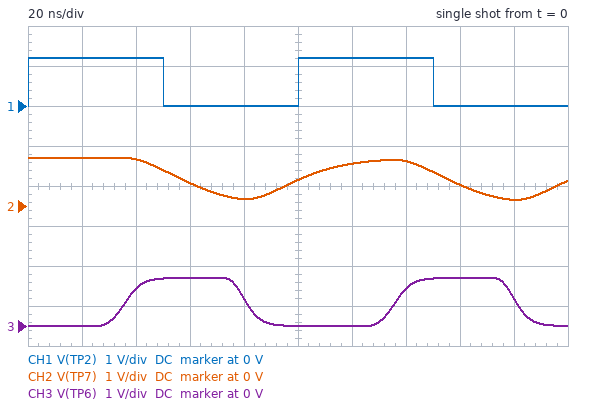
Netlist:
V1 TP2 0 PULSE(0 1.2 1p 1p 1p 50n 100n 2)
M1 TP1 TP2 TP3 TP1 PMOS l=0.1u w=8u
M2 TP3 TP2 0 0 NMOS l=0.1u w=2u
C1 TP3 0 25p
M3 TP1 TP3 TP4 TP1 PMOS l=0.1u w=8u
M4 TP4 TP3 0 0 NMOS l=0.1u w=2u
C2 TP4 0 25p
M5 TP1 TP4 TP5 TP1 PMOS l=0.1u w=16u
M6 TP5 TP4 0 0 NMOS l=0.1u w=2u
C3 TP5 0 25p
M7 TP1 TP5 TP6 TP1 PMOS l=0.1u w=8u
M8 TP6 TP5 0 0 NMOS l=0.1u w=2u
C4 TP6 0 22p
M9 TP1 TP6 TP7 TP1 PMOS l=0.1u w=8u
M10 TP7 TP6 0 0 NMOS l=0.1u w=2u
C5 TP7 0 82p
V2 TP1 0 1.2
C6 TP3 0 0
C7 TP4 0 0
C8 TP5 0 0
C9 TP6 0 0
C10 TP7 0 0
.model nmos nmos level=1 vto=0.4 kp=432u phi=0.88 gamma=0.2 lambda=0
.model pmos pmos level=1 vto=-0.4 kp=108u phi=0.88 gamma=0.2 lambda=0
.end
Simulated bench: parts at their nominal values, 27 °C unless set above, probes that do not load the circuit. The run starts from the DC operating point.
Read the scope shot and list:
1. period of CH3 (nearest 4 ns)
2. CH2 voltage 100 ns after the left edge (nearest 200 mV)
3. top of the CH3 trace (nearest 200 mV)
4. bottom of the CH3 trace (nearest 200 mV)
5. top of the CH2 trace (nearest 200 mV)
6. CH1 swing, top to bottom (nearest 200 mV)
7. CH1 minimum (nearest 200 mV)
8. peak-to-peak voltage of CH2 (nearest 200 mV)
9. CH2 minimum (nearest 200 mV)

100 ns
600 mV
1.2 V
0 V
1.2 V
1.2 V
0 V
1.0 V
200 mV
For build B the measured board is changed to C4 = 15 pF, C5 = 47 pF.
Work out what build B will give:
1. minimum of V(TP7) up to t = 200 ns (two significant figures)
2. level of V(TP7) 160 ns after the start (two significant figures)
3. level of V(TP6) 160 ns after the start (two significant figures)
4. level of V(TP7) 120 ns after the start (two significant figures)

13 mV
150 mV
1.2 V
1.2 V
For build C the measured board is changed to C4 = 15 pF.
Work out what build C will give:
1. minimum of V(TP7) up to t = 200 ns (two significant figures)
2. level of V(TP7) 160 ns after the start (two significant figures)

130 mV
440 mV
